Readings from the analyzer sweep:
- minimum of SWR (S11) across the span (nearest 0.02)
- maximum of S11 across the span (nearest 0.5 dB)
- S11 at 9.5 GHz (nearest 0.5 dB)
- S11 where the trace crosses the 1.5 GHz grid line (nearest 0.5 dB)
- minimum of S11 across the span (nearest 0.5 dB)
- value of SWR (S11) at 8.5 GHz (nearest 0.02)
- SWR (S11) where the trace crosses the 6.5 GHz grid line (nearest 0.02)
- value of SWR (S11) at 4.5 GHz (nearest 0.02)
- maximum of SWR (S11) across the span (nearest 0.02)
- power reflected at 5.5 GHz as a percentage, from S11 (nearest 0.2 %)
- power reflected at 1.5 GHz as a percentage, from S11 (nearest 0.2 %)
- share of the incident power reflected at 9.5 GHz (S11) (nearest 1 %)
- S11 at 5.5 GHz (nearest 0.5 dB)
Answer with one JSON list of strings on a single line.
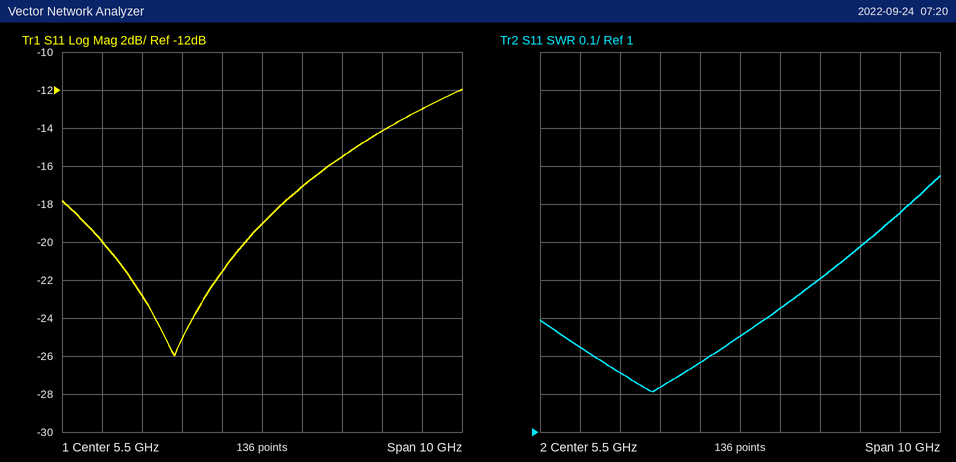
["1.10", "-12.0 dB", "-13.0 dB", "-20.0 dB", "-26.0 dB", "1.48", "1.32", "1.18", "1.68", "1.2 %", "1.0 %", "5 %", "-19.0 dB"]
